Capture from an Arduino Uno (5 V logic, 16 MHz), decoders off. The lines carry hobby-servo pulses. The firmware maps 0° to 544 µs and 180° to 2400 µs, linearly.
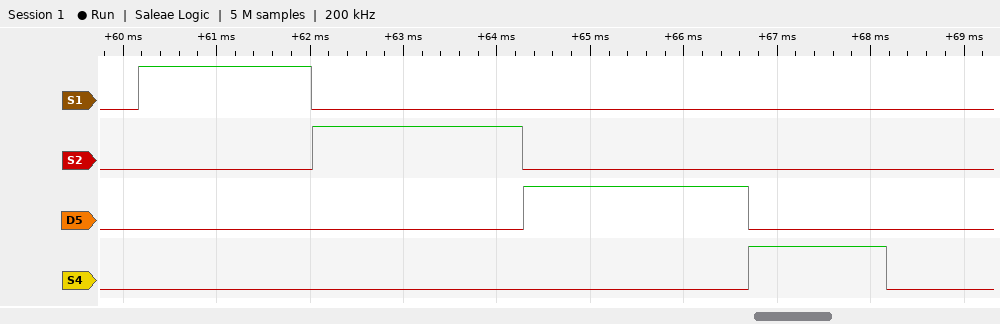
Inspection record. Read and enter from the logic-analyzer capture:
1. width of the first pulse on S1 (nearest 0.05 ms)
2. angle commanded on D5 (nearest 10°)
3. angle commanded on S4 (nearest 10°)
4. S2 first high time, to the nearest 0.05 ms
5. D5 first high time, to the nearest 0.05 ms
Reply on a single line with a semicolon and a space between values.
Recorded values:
1.85 ms; 180°; 90°; 2.25 ms; 2.40 ms
